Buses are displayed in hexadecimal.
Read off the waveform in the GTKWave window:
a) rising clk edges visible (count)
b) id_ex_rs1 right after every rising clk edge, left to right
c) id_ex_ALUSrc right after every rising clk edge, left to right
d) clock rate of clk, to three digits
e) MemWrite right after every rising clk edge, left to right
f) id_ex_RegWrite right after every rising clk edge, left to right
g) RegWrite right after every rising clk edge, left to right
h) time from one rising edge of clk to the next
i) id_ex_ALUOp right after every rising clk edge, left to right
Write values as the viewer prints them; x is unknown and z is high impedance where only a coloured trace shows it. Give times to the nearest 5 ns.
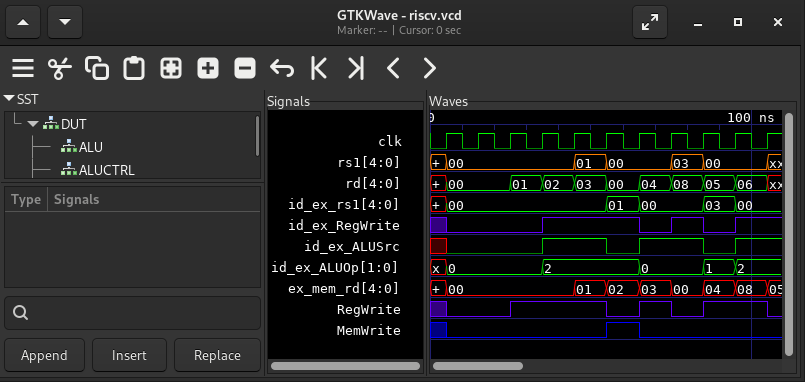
11
00, 00, 00, 00, 00, 01, 00, 00, 03, 00, 00
0 0 0 1 1 0 1 1 0 1 1
100 MHz
0 0 0 0 0 1 0 0 0 0 0
0 0 0 1 1 1 0 1 0 1 1
0 0 1 1 1 0 1 0 1 1 0
10 ns
0, 0, 0, 2, 2, 2, 0, 0, 1, 2, 2
